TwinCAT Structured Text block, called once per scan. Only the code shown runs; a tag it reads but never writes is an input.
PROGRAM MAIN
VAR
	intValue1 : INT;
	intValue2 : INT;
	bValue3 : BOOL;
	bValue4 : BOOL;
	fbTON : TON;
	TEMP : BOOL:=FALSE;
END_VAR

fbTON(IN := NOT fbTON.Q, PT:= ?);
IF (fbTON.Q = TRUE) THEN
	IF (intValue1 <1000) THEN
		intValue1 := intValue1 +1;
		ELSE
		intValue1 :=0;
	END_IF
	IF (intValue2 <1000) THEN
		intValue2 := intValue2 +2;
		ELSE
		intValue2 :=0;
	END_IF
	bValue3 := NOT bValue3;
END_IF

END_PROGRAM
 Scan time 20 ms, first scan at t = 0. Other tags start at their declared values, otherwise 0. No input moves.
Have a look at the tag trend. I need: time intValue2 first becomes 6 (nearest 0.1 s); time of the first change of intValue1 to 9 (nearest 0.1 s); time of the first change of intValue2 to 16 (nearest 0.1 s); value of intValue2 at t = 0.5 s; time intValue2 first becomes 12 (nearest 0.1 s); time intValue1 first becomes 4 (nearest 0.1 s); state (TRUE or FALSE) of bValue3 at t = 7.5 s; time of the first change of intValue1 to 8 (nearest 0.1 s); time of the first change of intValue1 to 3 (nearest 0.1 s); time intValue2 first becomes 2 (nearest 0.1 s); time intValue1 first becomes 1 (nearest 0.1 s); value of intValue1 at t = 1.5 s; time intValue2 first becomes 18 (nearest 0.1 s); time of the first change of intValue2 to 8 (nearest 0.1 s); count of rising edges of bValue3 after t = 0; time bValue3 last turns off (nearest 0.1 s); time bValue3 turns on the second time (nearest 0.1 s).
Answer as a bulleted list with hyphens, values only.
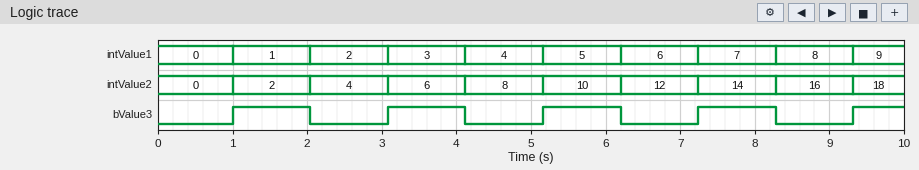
- 3.1 s
- 9.3 s
- 8.3 s
- 0
- 6.2 s
- 4.1 s
- TRUE
- 8.3 s
- 3.1 s
- 1.0 s
- 1.0 s
- 1
- 9.3 s
- 4.1 s
- 5
- 8.3 s
- 3.1 s
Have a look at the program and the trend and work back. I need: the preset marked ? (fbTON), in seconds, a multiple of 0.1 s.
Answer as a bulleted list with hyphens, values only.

- 1.0 s
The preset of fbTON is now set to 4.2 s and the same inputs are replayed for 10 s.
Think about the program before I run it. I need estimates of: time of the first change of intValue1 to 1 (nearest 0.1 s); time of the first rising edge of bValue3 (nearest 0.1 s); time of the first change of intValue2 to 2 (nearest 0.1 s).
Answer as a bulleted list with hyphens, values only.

- 4.2 s
- 4.2 s
- 4.2 s
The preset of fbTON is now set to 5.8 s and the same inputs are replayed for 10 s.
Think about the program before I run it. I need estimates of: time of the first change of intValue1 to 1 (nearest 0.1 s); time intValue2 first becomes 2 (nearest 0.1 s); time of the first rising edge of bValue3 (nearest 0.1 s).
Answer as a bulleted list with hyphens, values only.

- 5.8 s
- 5.8 s
- 5.8 s
